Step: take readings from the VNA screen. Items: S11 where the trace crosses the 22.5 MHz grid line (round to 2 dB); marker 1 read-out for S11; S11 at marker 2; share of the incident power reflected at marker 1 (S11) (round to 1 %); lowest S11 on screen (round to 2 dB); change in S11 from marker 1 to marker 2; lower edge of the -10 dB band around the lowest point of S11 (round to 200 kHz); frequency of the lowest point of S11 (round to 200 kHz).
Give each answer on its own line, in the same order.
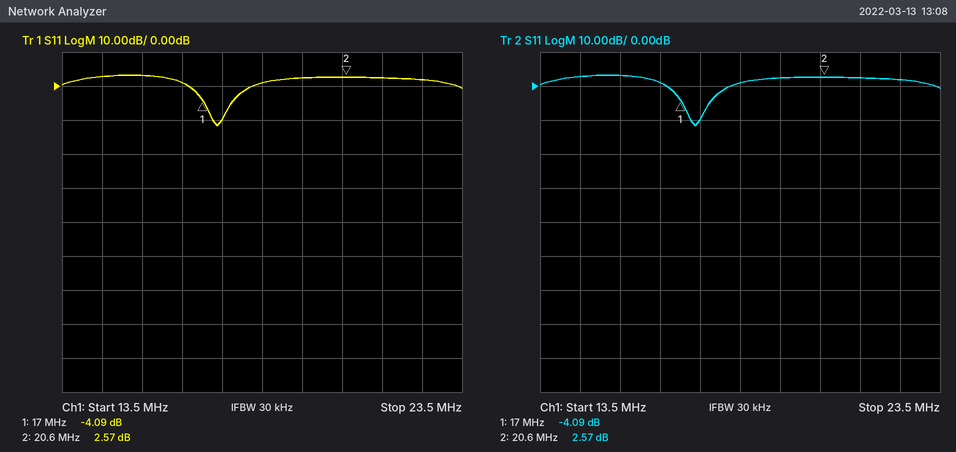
2 dB
-4.09 dB
2.57 dB
39 %
-12 dB
6.66 dB
17.2 MHz
17.4 MHz
